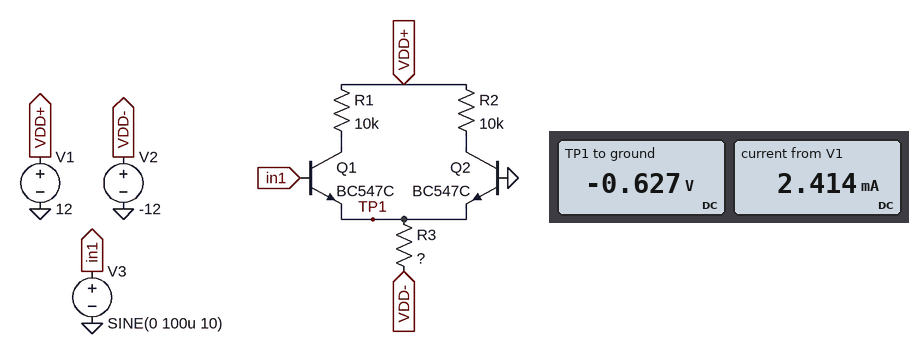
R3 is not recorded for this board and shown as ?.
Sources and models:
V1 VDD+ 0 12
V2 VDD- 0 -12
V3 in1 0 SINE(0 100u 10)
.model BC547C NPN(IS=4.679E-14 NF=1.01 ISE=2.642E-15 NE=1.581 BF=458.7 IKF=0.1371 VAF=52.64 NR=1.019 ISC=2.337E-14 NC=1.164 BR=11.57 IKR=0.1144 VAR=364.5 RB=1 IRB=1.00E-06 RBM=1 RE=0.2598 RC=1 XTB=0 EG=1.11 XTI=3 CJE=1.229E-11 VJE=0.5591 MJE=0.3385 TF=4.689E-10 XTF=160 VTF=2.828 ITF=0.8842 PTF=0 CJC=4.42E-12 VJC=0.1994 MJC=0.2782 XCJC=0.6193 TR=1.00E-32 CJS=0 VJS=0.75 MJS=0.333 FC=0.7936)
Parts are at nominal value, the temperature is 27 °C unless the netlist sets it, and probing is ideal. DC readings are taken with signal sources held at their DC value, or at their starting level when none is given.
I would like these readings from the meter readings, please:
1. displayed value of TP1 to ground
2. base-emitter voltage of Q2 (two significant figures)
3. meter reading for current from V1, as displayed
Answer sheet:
-0.627 V
630 mV
2.414 mA
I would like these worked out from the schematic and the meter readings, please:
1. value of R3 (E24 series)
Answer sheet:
4.7 kΩ
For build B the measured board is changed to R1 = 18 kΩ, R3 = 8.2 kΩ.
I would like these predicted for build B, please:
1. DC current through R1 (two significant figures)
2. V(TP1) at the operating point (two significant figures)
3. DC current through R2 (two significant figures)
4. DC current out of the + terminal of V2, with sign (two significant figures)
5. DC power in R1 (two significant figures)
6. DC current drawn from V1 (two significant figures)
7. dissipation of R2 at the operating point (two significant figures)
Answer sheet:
660 µA
-610 mV
720 µA
-1.4 mA
7.9 mW
1.4 mA
5.2 mW
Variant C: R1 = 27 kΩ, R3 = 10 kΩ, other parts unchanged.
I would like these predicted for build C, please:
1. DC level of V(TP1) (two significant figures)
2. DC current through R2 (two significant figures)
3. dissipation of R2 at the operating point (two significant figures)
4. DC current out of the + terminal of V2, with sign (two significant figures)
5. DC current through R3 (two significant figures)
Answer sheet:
-610 mV
660 µA
4.3 mW
-1.1 mA
1.1 mA
